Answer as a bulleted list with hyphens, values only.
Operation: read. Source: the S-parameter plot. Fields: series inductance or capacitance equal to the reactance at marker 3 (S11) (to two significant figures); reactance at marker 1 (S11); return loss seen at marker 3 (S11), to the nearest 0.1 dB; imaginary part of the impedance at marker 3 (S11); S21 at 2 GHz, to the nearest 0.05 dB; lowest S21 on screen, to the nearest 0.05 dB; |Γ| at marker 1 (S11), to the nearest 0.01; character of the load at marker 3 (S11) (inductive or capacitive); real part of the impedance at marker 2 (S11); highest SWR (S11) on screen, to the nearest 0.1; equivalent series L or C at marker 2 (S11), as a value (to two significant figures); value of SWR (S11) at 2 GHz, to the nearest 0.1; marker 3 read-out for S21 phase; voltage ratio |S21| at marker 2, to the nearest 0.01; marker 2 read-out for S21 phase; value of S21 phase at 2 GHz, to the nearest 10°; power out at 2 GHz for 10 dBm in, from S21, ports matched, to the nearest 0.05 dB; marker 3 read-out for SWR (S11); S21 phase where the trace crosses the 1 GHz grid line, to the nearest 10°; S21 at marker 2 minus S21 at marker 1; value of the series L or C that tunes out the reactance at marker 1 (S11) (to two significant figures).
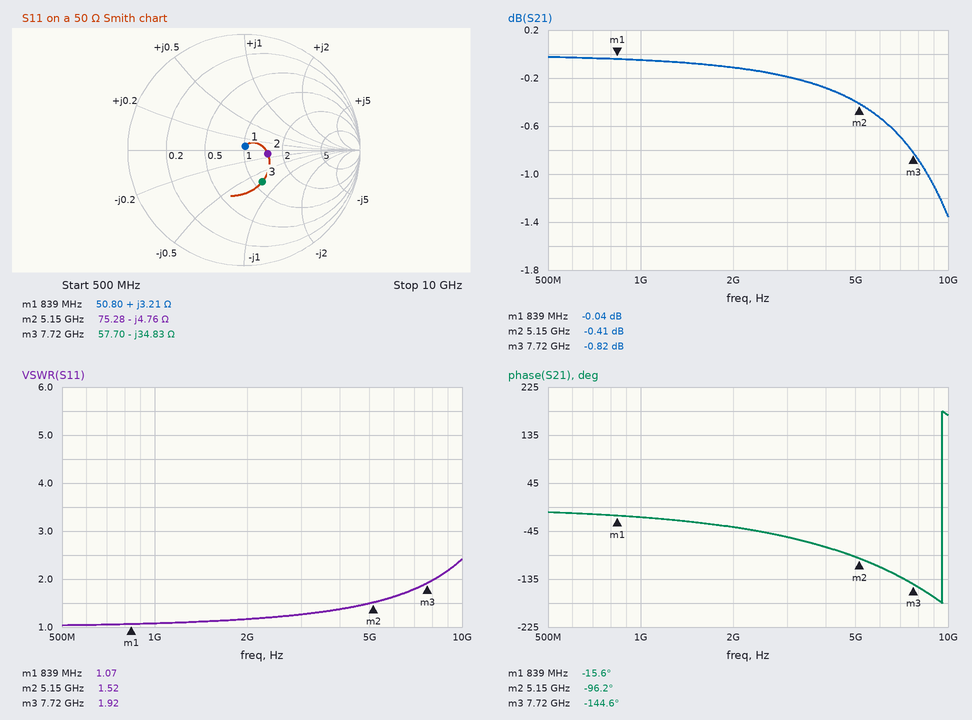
- 590 fF
- +3.21 Ω
- 10.0 dB
- -34.83 Ω
- -0.10 dB
- -1.35 dB
- 0.03
- capacitive
- 75.28 Ω
- 2.4
- 6.5 pF
- 1.2
- -144.6°
- 0.95
- -96.2°
- -40°
- 9.90 dBm
- 1.92
- -20°
- -0.37 dB
- 59 pF
